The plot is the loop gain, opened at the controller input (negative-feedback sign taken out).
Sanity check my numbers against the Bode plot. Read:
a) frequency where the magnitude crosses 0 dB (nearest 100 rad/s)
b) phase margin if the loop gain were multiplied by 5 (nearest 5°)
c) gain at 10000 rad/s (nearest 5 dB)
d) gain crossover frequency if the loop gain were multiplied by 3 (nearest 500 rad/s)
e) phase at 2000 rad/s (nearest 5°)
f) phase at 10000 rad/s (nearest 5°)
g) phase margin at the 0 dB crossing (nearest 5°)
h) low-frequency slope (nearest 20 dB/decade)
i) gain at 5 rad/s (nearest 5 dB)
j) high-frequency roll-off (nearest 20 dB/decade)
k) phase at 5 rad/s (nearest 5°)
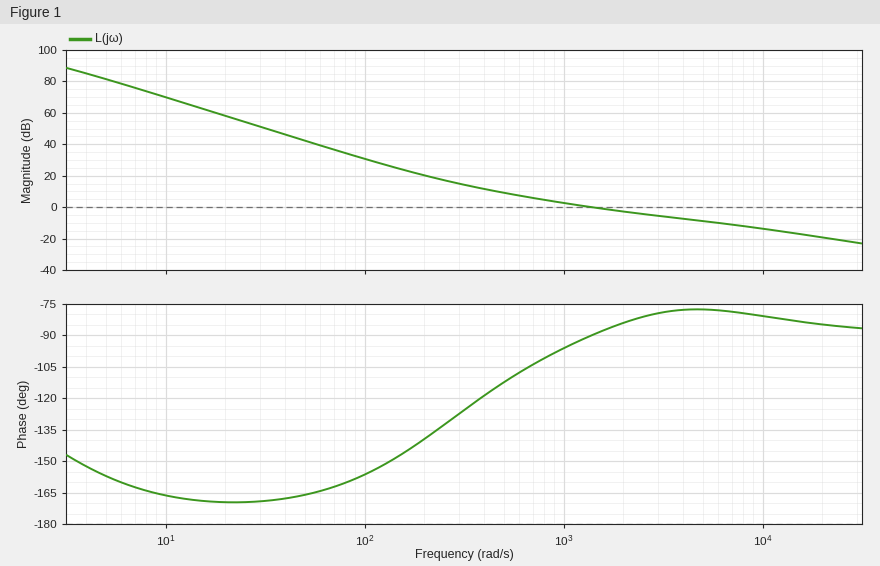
1400 rad/s
100°
-15 dB
5500 rad/s
-85°
-80°
90°
-40 dB/decade
80 dB
-20 dB/decade
-155°
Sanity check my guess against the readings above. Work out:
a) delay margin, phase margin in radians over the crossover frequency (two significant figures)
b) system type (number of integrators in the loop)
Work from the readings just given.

0.0011 s
2
